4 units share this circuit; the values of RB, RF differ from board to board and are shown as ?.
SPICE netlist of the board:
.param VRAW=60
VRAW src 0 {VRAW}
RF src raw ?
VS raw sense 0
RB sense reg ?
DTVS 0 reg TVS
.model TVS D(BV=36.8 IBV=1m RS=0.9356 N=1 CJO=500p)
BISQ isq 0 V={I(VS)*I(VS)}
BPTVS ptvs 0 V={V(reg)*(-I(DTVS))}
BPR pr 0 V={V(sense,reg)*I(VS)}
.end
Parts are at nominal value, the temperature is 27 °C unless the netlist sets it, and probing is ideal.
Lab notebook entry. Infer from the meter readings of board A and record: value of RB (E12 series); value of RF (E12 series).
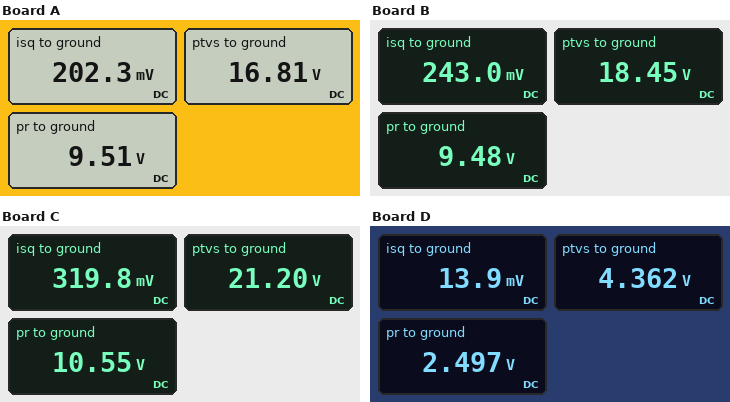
47 Ω
3.3 Ω
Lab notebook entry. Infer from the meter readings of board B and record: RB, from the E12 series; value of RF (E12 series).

39 Ω
6.8 Ω
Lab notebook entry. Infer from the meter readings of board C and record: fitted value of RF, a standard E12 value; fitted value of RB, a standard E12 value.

6.8 Ω
33 Ω
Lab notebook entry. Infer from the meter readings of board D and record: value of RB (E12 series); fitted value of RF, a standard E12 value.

180 Ω
15 Ω
